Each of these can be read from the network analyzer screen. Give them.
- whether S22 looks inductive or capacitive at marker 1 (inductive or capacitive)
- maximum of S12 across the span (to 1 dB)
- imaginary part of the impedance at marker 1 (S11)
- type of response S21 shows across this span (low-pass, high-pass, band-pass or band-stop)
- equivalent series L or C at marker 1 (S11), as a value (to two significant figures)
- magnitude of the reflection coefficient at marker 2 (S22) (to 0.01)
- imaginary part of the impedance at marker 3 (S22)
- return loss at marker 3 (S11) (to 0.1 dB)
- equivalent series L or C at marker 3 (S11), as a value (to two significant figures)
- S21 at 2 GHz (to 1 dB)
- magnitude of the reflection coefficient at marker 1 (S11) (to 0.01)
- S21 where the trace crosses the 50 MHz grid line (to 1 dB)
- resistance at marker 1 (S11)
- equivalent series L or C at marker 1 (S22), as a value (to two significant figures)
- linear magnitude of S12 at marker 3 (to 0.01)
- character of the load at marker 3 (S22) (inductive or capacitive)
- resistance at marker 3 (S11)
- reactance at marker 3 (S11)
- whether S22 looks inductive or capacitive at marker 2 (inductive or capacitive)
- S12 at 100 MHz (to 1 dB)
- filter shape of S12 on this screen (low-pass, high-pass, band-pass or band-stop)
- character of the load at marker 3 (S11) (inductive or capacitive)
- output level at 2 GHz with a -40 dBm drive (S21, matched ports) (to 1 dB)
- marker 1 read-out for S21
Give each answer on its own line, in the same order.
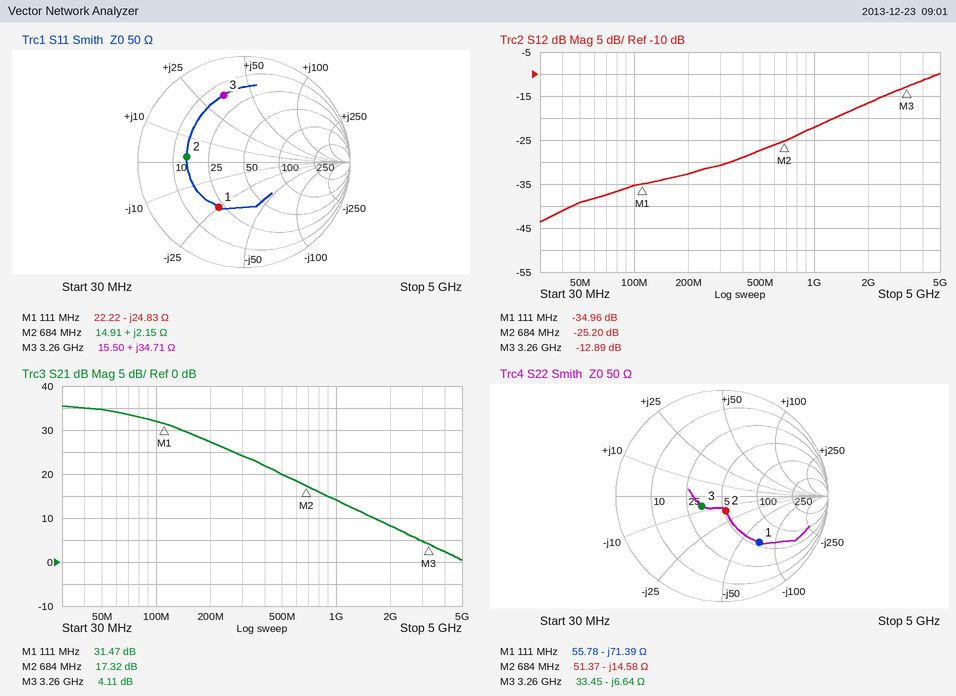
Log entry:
capacitive
-10 dB
-24.83 Ω
low-pass
58 pF
0.14
-6.64 Ω
3.6 dB
1.7 nH
8 dB
0.49
35 dB
22.22 Ω
20 pF
0.23
capacitive
15.50 Ω
+34.71 Ω
capacitive
-35 dB
high-pass
inductive
-32 dBm
31.47 dB
